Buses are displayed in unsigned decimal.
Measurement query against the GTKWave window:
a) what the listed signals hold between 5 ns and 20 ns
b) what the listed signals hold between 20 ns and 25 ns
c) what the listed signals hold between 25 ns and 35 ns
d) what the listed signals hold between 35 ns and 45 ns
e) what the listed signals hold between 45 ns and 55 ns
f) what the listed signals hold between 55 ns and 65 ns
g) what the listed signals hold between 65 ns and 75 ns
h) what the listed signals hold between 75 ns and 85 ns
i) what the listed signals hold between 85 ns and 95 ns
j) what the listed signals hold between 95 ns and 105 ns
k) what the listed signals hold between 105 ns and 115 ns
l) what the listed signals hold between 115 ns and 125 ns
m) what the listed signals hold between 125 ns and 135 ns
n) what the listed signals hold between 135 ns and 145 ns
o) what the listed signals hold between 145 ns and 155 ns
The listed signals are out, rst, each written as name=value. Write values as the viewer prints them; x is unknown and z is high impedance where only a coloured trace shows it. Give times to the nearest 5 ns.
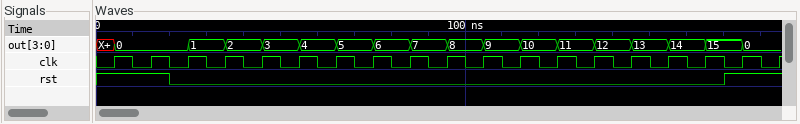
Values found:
out=0, rst=1
out=0, rst=0
out=1, rst=0
out=2, rst=0
out=3, rst=0
out=4, rst=0
out=5, rst=0
out=6, rst=0
out=7, rst=0
out=8, rst=0
out=9, rst=0
out=10, rst=0
out=11, rst=0
out=12, rst=0
out=13, rst=0
